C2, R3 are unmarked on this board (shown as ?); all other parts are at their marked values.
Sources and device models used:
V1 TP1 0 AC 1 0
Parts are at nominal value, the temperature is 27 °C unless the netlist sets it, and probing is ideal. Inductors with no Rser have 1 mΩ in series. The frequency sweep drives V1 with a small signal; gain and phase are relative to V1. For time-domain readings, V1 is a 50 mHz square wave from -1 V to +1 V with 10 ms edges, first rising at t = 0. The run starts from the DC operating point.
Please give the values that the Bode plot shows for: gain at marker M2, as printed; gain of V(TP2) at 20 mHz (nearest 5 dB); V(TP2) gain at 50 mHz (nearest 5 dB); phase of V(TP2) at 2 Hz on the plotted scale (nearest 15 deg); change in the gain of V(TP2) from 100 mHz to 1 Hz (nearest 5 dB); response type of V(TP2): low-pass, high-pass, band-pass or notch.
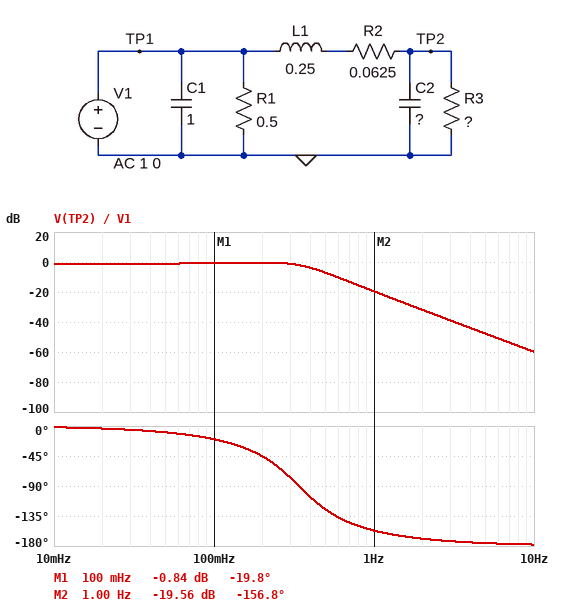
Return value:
-19.56 dB
0 dB
0 dB
-165 deg
-20 dB
low-pass
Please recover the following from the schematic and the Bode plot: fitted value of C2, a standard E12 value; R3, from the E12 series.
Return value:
1 F
0.47 Ω
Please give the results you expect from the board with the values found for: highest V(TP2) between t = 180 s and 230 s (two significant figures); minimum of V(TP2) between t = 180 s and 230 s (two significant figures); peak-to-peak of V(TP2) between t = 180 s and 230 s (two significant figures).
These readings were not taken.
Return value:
1.1 V
-1.1 V
2.2 V
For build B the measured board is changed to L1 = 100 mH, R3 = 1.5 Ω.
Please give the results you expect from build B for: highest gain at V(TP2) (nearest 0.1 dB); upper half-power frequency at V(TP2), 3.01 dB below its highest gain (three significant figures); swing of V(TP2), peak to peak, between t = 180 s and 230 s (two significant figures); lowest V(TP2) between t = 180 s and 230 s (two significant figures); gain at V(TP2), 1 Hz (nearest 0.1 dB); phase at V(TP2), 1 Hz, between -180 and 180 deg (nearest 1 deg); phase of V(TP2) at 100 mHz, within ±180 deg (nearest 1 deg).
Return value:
7.7 dB
589 mHz
3.9 V
-2.0 V
-9.6 dB
-164 deg
-5 deg
